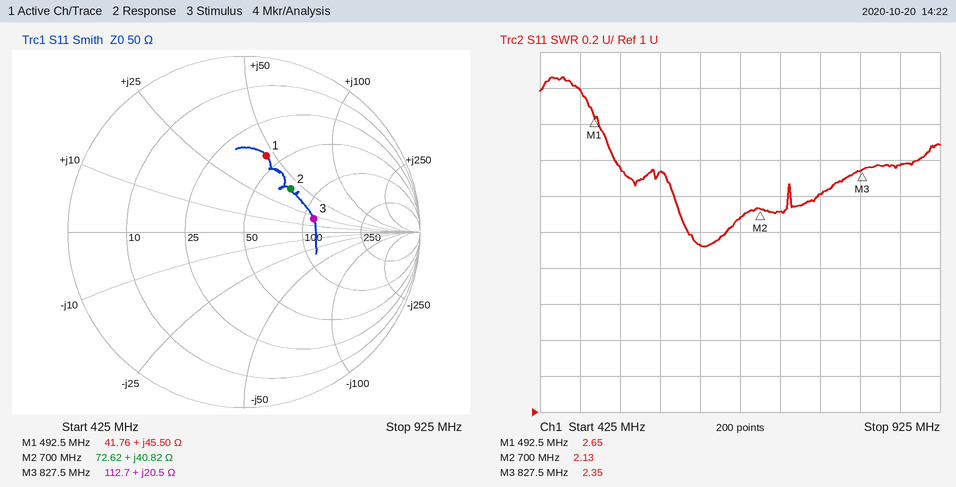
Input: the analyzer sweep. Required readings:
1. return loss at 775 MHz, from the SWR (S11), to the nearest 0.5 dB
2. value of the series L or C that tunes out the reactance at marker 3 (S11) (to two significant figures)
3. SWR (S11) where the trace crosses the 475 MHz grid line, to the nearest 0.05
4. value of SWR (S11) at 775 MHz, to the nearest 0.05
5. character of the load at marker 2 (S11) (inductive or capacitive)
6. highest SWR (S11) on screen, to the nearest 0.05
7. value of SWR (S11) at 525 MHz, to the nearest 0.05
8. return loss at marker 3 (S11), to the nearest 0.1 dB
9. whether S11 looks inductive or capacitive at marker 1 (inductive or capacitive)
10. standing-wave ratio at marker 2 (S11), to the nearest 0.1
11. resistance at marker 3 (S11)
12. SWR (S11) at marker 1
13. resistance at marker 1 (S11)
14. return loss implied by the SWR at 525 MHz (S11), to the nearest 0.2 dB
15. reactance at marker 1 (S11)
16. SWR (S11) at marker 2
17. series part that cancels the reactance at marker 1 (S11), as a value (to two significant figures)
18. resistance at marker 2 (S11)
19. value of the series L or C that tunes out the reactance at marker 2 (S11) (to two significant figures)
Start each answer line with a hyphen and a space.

- 8.5 dB
- 9.4 pF
- 2.80
- 2.20
- inductive
- 2.85
- 2.35
- 7.9 dB
- inductive
- 2.1
- 112.7 Ω
- 2.65
- 41.76 Ω
- 7.8 dB
- +45.50 Ω
- 2.13
- 7.1 pF
- 72.62 Ω
- 5.6 pF
